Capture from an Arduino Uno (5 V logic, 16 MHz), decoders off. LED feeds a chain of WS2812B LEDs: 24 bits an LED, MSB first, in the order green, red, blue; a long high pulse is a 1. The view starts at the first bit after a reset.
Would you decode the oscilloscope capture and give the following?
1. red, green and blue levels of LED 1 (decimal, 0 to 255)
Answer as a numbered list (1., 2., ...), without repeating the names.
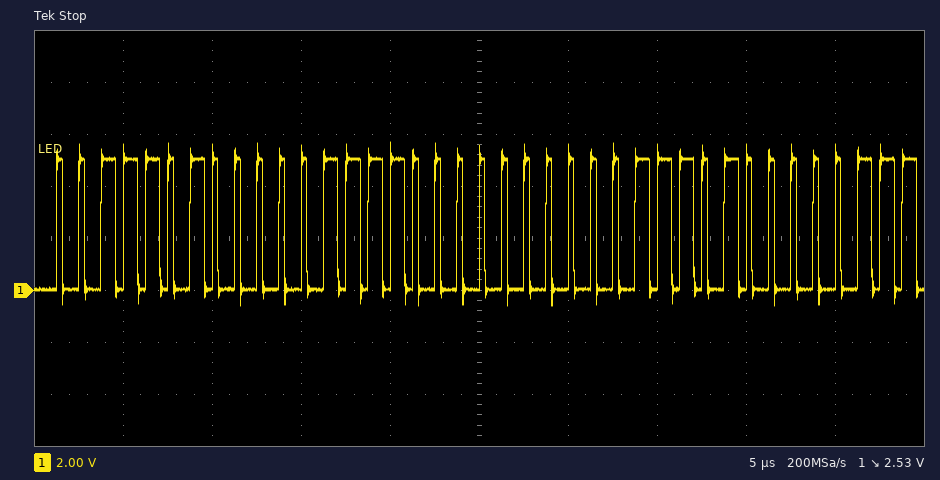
1. 15, 58, 0
